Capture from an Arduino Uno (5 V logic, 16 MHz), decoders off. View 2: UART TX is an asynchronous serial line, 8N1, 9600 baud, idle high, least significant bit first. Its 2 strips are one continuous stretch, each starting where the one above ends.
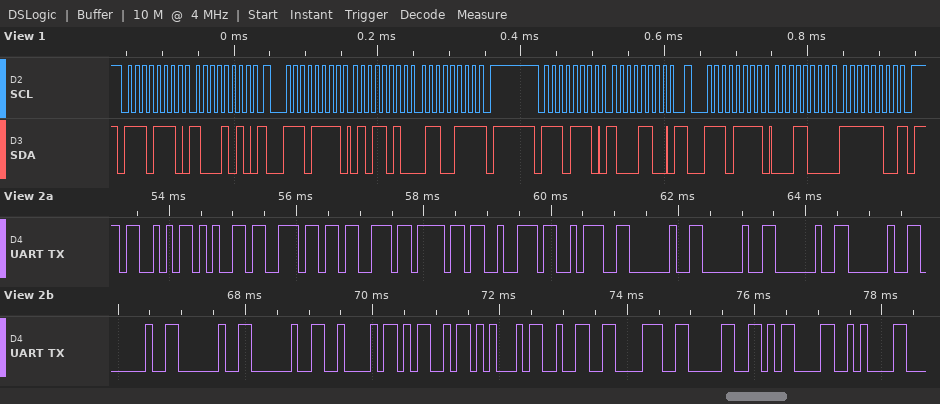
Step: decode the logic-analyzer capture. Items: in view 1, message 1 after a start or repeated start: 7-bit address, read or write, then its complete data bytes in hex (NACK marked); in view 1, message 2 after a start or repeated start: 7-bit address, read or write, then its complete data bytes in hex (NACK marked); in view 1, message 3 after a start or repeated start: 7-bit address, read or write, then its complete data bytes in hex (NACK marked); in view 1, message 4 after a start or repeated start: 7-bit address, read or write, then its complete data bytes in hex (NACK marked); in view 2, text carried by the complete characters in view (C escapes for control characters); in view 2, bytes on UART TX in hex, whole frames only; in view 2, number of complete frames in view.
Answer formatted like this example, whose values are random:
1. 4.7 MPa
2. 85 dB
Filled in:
1. 0x77 write: 8A
2. 0x77 read: 5A 67 NACK
3. 0x77 write: 8C
4. 0x77 read: 18 FC NACK
5. "Sensor:       BME280\r\n"
6. 53 65 6E 73 6F 72 3A 20 20 20 20 20 20 20 42 4D 45 32 38 30 0D 0A
7. 22
